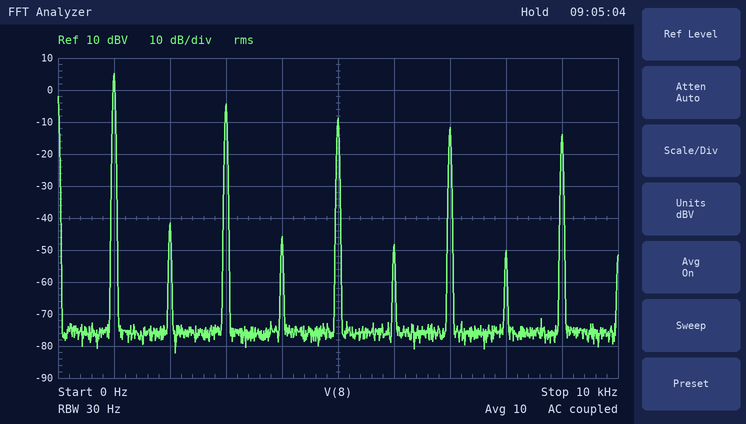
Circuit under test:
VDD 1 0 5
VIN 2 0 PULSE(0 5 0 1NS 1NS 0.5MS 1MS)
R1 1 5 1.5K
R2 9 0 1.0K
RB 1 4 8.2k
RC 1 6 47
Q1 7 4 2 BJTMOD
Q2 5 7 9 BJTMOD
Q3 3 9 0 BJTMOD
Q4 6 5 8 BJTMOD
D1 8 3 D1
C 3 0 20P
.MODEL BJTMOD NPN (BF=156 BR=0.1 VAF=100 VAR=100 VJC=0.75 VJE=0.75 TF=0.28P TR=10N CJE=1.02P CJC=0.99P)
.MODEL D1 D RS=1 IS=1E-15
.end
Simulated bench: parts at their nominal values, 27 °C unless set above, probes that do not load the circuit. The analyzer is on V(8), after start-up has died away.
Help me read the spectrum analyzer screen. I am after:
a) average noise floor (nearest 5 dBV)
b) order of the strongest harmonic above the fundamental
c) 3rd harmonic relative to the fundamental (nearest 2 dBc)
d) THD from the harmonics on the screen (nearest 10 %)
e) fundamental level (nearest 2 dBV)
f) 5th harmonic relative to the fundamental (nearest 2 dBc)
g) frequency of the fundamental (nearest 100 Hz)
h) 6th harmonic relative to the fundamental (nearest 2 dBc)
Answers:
-75 dBV
3
-10 dBc
40 %
6 dBV
-14 dBc
1.0 kHz
-54 dBc
